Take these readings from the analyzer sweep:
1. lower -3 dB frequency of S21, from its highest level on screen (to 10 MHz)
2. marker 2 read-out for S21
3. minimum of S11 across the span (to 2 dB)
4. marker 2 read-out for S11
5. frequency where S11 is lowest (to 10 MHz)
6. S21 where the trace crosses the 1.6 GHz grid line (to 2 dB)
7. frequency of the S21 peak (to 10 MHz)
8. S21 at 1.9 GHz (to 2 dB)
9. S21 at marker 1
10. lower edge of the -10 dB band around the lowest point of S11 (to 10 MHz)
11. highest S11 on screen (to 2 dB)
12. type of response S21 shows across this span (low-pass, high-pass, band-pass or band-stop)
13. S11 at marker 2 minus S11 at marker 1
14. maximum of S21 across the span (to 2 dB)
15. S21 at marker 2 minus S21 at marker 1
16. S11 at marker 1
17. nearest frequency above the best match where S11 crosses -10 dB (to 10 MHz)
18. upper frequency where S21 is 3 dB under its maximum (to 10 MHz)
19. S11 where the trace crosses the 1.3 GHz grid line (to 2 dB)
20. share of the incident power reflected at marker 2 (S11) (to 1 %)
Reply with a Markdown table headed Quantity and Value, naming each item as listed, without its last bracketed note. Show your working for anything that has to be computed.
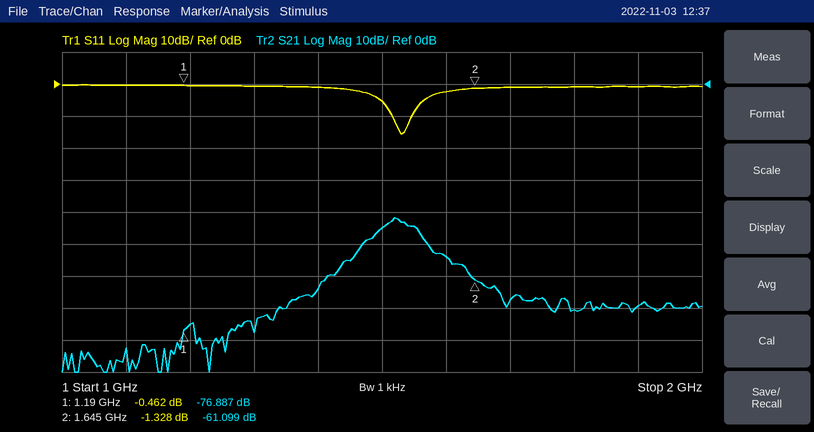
| Quantity | Value |
|---|---|
| lower -3 dB frequency of S21, from its highest level on screen | 1.50 GHz |
| marker 2 read-out for S21 | -61.099 dB |
| minimum of S11 across the span | -16 dB |
| marker 2 read-out for S11 | -1.328 dB |
| frequency where S11 is lowest | 1.53 GHz |
| S21 where the trace crosses the 1.6 GHz grid line | -54 dB |
| frequency of the S21 peak | 1.52 GHz |
| S21 at 1.9 GHz | -70 dB |
| S21 at marker 1 | -76.887 dB |
| lower edge of the -10 dB band around the lowest point of S11 | 1.52 GHz |
| highest S11 on screen | 0 dB |
| type of response S21 shows across this span | band-pass |
| S11 at marker 2 minus S11 at marker 1 | -1.328 − (-0.462) = -0.866 dB |
| maximum of S21 across the span | -42 dB |
| S21 at marker 2 minus S21 at marker 1 | -61.099 − (-76.887) = 15.788 dB |
| S11 at marker 1 | -0.462 dB |
| nearest frequency above the best match where S11 crosses -10 dB | 1.55 GHz |
| upper frequency where S21 is 3 dB under its maximum | 1.55 GHz |
| S11 where the trace crosses the 1.3 GHz grid line | 0 dB |
| share of the incident power reflected at marker 2 (S11) | 10^(-1.328/10) ≈ 74 % |
